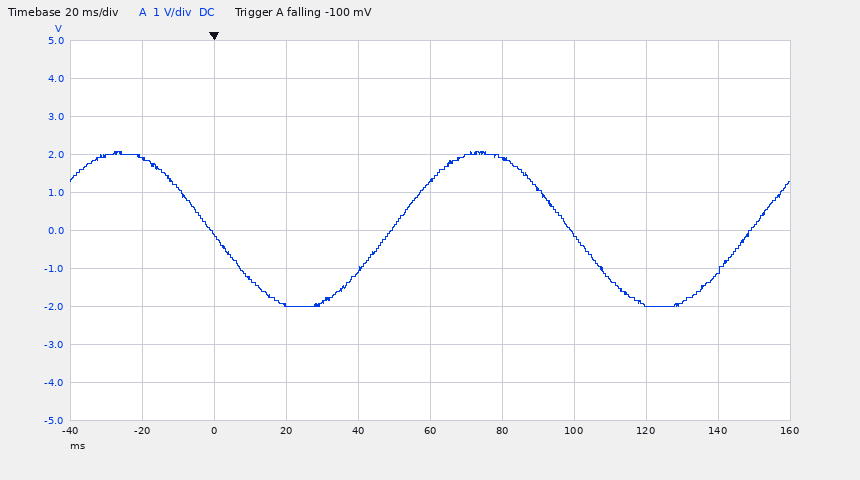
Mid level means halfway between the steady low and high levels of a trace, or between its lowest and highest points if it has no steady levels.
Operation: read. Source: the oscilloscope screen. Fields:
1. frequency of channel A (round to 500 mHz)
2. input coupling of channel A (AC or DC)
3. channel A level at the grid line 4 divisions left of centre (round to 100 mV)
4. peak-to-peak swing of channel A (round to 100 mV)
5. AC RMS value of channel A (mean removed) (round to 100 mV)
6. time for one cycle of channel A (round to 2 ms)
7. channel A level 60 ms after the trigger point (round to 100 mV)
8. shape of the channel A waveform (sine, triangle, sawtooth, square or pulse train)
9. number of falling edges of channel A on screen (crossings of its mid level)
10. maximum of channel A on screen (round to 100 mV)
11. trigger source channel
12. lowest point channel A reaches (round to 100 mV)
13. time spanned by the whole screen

10.0 Hz
DC
1.9 V
4.1 V
1.4 V
100 ms
1.3 V
sine
2
2.1 V
channel A
-2.0 V
200 ms
